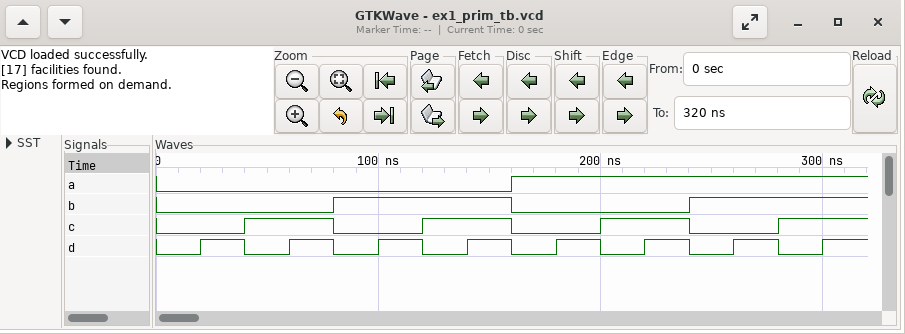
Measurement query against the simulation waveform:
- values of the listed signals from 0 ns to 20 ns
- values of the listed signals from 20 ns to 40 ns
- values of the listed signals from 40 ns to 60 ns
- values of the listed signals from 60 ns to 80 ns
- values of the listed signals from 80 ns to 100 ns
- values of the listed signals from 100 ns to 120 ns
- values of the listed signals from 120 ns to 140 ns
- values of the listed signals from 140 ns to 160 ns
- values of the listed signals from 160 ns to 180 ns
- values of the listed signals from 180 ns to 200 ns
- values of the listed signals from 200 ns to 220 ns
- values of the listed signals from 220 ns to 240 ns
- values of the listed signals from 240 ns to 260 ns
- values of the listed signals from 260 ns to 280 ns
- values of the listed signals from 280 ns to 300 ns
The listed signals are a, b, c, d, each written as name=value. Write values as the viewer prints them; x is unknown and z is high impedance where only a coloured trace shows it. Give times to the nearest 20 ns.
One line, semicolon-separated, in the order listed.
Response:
a=0, b=0, c=0, d=0; a=0, b=0, c=0, d=1; a=0, b=0, c=1, d=0; a=0, b=0, c=1, d=1; a=0, b=1, c=0, d=0; a=0, b=1, c=0, d=1; a=0, b=1, c=1, d=0; a=0, b=1, c=1, d=1; a=1, b=0, c=0, d=0; a=1, b=0, c=0, d=1; a=1, b=0, c=1, d=0; a=1, b=0, c=1, d=1; a=1, b=1, c=0, d=0; a=1, b=1, c=0, d=1; a=1, b=1, c=1, d=0
